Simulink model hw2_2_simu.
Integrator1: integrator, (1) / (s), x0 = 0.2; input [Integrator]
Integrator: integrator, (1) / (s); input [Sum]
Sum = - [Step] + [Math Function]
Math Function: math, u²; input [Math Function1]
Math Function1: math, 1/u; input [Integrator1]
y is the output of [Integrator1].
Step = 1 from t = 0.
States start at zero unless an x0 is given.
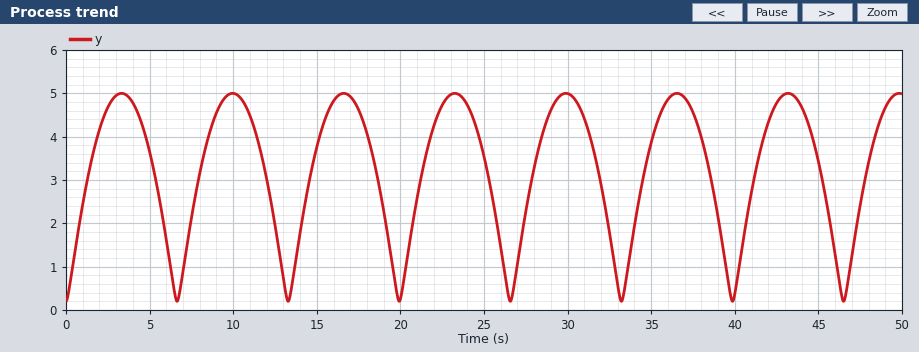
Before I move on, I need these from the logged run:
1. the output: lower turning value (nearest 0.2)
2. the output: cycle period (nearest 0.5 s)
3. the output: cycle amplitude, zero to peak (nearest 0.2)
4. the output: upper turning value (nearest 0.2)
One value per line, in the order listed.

0.2
6.5 s
2.4
5.0
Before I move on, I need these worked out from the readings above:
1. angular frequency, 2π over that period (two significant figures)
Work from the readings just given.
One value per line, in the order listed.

0.97 rad/s
